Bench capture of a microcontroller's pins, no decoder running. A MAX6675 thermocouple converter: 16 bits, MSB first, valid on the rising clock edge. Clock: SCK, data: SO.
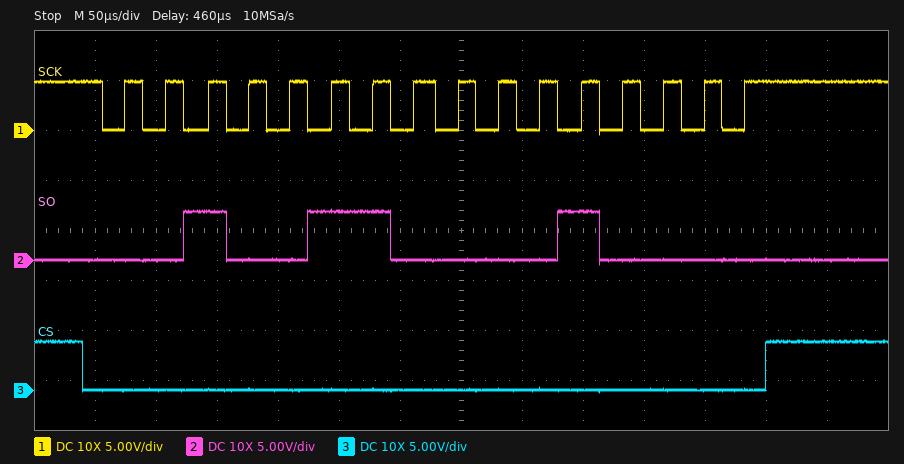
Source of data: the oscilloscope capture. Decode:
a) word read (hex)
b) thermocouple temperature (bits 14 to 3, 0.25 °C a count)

0x2610
304.50 °C
